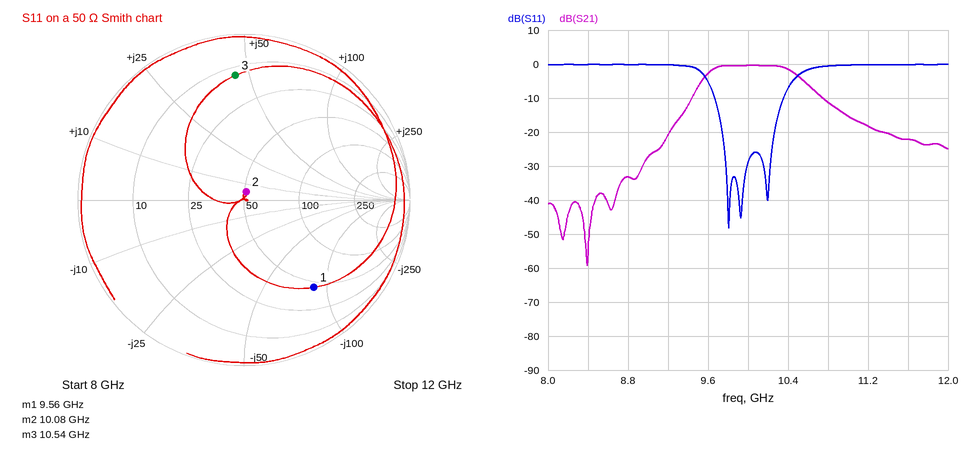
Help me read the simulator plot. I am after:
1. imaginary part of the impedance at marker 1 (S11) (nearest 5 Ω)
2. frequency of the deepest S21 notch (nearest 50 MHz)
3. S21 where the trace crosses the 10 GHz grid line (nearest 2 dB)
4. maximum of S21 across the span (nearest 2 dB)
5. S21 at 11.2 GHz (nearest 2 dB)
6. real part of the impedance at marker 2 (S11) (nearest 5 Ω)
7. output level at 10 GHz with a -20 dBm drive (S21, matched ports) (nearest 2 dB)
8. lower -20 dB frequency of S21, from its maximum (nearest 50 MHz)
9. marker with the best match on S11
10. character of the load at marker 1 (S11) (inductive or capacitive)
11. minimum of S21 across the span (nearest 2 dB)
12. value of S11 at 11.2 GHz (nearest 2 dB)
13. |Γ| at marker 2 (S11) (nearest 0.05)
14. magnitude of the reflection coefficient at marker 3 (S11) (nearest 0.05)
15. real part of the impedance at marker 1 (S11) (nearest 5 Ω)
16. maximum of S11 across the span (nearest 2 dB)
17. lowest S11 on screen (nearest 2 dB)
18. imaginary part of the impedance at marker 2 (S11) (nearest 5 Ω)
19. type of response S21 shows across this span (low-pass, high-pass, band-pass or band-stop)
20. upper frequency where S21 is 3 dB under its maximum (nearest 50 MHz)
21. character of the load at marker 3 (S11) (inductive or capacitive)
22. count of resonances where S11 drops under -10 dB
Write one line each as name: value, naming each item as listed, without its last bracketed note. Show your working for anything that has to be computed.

imaginary part of the impedance at marker 1 (S11): -85 Ω
frequency of the deepest S21 notch: 8.40 GHz
S21 where the trace crosses the 10 GHz grid line: 0 dB
maximum of S21 across the span: 0 dB
S21 at 11.2 GHz: -18 dB
real part of the impedance at marker 2 (S11): 50 Ω
output level at 10 GHz with a -20 dBm drive (S21, matched ports): -20 dBm + (0 dB) = -20 dBm
lower -20 dB frequency of S21, from its maximum: 9.20 GHz
marker with the best match on S11: marker 2
character of the load at marker 1 (S11): capacitive
minimum of S21 across the span: -60 dB
value of S11 at 11.2 GHz: 0 dB
|Γ| at marker 2 (S11): 0.05
magnitude of the reflection coefficient at marker 3 (S11): 0.75
real part of the impedance at marker 1 (S11): 45 Ω
maximum of S11 across the span: 0 dB
lowest S11 on screen: -48 dB
imaginary part of the impedance at marker 2 (S11): +5 Ω
type of response S21 shows across this span: band-pass
upper frequency where S21 is 3 dB under its maximum: 10.50 GHz
character of the load at marker 3 (S11): inductive
count of resonances where S11 drops under -10 dB: 3
